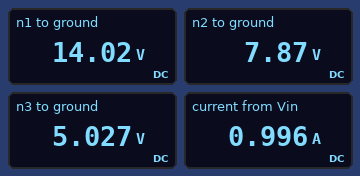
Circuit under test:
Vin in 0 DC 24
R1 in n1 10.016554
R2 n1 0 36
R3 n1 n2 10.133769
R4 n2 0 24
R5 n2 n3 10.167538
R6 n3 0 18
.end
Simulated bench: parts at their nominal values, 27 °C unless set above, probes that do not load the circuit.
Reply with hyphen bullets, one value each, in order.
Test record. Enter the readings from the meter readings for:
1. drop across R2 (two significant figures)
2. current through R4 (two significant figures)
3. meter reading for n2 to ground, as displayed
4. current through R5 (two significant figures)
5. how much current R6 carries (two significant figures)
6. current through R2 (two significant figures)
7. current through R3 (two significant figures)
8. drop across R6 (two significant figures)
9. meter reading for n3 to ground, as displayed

- 14 V
- 330 mA
- 7.87 V
- 280 mA
- 280 mA
- 390 mA
- 610 mA
- 5.0 V
- 5.027 V
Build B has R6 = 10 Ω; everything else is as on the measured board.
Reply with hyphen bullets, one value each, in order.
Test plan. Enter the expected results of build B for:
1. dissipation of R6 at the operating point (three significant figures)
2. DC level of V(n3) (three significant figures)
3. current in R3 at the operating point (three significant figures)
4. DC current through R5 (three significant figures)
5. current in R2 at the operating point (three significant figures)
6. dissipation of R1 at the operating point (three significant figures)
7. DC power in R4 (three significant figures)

- 1.24 W
- 3.53 V
- 649 mA
- 353 mA
- 380 mA
- 10.6 W
- 2.11 W
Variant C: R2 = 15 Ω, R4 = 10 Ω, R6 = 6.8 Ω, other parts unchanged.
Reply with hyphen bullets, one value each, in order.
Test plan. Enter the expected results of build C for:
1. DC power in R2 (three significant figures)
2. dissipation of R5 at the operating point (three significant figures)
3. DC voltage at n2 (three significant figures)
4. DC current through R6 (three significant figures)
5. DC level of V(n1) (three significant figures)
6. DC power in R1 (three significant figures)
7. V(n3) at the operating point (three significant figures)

- 7.40 W
- 575 mW
- 4.04 V
- 238 mA
- 10.5 V
- 18.1 W
- 1.62 V
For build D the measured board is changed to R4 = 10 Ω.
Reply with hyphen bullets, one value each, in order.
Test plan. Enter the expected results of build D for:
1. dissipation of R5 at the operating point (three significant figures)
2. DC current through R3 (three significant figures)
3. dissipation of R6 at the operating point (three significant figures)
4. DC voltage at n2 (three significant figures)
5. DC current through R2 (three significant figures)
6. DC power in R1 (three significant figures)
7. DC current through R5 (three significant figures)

- 383 mW
- 741 mA
- 678 mW
- 5.47 V
- 360 mA
- 12.1 W
- 194 mA
